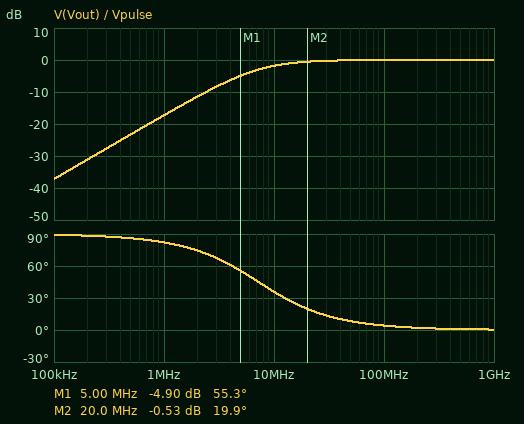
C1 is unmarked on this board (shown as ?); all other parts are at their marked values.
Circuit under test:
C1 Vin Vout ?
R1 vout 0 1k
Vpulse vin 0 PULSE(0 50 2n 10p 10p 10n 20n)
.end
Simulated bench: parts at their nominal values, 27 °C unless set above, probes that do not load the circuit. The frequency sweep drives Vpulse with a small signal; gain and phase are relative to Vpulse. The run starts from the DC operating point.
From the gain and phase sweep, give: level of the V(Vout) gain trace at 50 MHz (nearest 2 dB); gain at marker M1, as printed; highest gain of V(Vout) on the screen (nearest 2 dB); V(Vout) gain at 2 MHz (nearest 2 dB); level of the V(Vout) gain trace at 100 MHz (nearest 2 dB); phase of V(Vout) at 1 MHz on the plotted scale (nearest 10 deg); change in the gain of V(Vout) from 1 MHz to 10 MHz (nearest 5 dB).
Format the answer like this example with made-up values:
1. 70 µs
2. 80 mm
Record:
1. 0 dB
2. -4.90 dB
3. 0 dB
4. -12 dB
5. 0 dB
6. 80 deg
7. 15 dB
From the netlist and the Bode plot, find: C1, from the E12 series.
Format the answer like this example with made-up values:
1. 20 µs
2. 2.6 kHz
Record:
1. 22 pF
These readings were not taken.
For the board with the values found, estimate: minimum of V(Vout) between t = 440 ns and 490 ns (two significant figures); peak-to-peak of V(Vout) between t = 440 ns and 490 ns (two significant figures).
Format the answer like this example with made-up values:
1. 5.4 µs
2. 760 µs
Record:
1. -31 V
2. 61 V
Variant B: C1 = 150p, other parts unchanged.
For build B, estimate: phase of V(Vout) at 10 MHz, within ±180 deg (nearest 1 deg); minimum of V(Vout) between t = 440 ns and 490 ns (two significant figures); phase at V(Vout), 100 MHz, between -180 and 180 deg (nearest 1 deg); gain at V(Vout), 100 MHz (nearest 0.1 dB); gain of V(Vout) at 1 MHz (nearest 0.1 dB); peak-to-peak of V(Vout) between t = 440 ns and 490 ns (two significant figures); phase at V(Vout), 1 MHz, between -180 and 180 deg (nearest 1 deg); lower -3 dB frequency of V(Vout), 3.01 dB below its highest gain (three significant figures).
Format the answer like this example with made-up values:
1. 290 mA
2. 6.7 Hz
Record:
1. 6 deg
2. -25 V
3. 1 deg
4. 0 dB
5. -3.3 dB
6. 52 V
7. 47 deg
8. 1.06 MHz
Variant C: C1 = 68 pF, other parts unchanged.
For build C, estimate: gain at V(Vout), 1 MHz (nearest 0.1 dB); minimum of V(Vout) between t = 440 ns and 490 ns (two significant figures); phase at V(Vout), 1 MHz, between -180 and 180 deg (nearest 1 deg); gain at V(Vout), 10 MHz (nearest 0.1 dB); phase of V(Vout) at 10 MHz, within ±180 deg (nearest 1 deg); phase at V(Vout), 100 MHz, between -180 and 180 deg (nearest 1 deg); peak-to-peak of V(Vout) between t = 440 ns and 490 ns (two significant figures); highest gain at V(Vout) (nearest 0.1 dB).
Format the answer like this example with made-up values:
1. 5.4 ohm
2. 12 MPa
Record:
1. -8.1 dB
2. -27 V
3. 67 deg
4. -0.2 dB
5. 13 deg
6. 1 deg
7. 54 V
8. 0 dB
